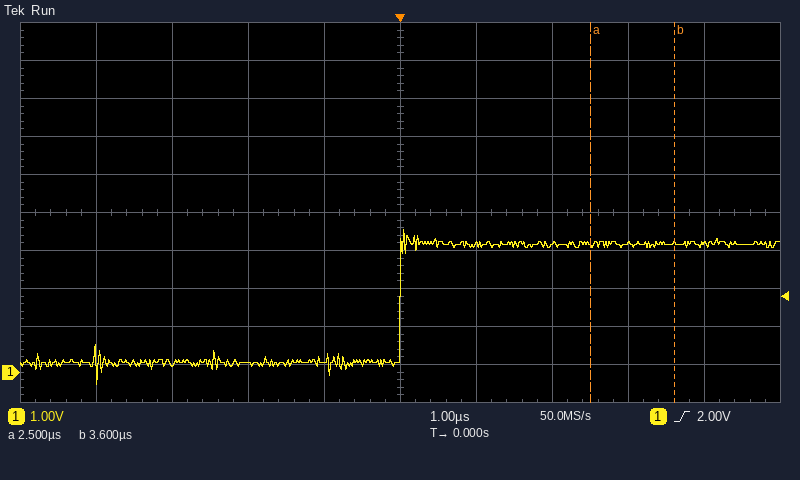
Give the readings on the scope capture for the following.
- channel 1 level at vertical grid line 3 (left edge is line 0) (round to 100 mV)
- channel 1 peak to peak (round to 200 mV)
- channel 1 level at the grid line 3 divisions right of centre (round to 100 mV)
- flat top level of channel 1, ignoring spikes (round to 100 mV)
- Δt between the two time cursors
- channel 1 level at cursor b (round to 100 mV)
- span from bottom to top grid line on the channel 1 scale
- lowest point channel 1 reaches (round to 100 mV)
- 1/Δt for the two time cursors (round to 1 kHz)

200 mV
4.0 V
3.4 V
3.4 V
1.1 µs
3.4 V
10 V
-300 mV
909 kHz
